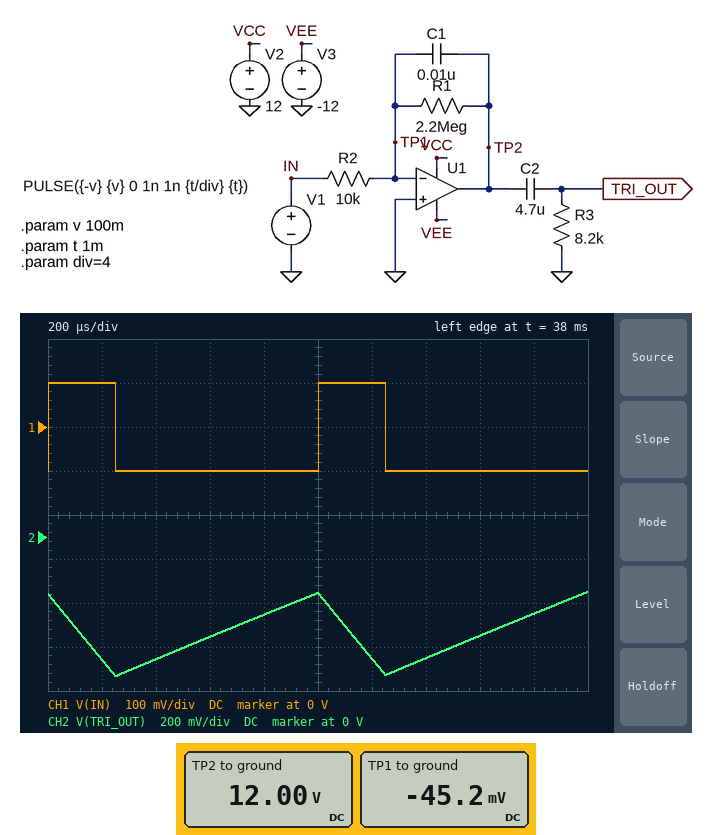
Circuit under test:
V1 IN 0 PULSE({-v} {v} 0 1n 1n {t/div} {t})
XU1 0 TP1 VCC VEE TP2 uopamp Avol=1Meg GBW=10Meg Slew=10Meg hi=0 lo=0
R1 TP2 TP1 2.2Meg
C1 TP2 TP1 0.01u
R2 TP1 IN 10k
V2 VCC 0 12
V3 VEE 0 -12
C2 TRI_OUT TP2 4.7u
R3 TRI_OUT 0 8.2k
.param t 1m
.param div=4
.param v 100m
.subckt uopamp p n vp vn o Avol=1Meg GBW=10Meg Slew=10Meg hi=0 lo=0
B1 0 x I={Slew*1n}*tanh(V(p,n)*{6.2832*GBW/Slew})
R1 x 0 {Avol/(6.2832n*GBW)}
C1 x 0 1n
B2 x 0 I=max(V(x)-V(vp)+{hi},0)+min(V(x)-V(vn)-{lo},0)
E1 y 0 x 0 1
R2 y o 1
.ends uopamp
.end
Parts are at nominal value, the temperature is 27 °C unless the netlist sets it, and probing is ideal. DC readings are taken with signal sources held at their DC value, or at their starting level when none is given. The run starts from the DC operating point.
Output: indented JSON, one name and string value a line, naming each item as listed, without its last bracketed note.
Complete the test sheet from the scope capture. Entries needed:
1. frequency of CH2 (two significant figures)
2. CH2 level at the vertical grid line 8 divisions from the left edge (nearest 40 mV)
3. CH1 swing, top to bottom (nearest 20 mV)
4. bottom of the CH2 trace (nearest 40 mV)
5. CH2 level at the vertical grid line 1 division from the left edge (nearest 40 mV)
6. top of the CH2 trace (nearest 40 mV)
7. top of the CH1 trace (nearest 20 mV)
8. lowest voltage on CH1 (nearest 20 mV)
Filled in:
{
  "frequency of CH2": "1.0 kHz",
  "CH2 level at the vertical grid line 8 divisions from the left edge": "-440 mV",
  "CH1 swing, top to bottom": "200 mV",
  "bottom of the CH2 trace": "-640 mV",
  "CH2 level at the vertical grid line 1 division from the left edge": "-560 mV",
  "top of the CH2 trace": "-240 mV",
  "top of the CH1 trace": "100 mV",
  "lowest voltage on CH1": "-100 mV"
}
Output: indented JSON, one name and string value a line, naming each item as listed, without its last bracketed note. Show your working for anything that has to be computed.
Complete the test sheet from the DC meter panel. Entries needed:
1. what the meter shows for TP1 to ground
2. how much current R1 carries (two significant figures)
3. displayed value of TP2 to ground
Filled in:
{
  "what the meter shows for TP1 to ground": "-45.2 mV",
  "how much current R1 carries": "(12 V - (-45.2 mV)) / 2.2 MΩ = 5.5 µA",
  "displayed value of TP2 to ground": "12.00 V"
}
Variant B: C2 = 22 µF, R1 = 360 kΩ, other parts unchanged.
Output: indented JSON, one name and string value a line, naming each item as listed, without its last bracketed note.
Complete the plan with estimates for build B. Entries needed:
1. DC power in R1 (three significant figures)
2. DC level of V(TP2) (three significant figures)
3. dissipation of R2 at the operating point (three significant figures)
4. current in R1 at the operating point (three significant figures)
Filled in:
{
  "DC power in R1": "36.0 µW",
  "DC level of V(TP2)": "3.60 V",
  "dissipation of R2 at the operating point": "1.00 µW",
  "current in R1 at the operating point": "10.0 µA"
}
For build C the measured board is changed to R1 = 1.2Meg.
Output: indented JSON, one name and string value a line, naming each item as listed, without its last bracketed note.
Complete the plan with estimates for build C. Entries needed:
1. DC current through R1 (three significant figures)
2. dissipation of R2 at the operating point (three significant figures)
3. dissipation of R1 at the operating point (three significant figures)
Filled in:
{
  "DC current through R1": "10.0 µA",
  "dissipation of R2 at the operating point": "1.00 µW",
  "dissipation of R1 at the operating point": "120 µW"
}
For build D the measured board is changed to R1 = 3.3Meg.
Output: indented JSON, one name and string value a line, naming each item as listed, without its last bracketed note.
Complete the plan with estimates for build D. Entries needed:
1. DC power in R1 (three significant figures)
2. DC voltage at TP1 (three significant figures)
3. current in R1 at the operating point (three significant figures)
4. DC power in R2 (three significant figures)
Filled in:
{
  "DC power in R1": "44.1 µW",
  "DC voltage at TP1": "-63.4 mV",
  "current in R1 at the operating point": "3.66 µA",
  "DC power in R2": "134 nW"
}
